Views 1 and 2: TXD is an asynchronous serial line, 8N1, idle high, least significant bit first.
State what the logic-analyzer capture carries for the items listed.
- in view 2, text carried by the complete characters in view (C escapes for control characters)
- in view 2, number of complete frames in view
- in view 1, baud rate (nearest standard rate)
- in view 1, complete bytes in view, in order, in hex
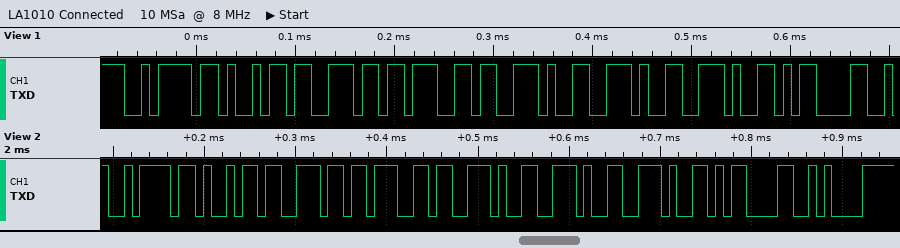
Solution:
"zing...\r\n"
9
115200 baud
0x7A 0x69 0x6E 0x67 0x2E 0x2E 0x2E 0x0D
